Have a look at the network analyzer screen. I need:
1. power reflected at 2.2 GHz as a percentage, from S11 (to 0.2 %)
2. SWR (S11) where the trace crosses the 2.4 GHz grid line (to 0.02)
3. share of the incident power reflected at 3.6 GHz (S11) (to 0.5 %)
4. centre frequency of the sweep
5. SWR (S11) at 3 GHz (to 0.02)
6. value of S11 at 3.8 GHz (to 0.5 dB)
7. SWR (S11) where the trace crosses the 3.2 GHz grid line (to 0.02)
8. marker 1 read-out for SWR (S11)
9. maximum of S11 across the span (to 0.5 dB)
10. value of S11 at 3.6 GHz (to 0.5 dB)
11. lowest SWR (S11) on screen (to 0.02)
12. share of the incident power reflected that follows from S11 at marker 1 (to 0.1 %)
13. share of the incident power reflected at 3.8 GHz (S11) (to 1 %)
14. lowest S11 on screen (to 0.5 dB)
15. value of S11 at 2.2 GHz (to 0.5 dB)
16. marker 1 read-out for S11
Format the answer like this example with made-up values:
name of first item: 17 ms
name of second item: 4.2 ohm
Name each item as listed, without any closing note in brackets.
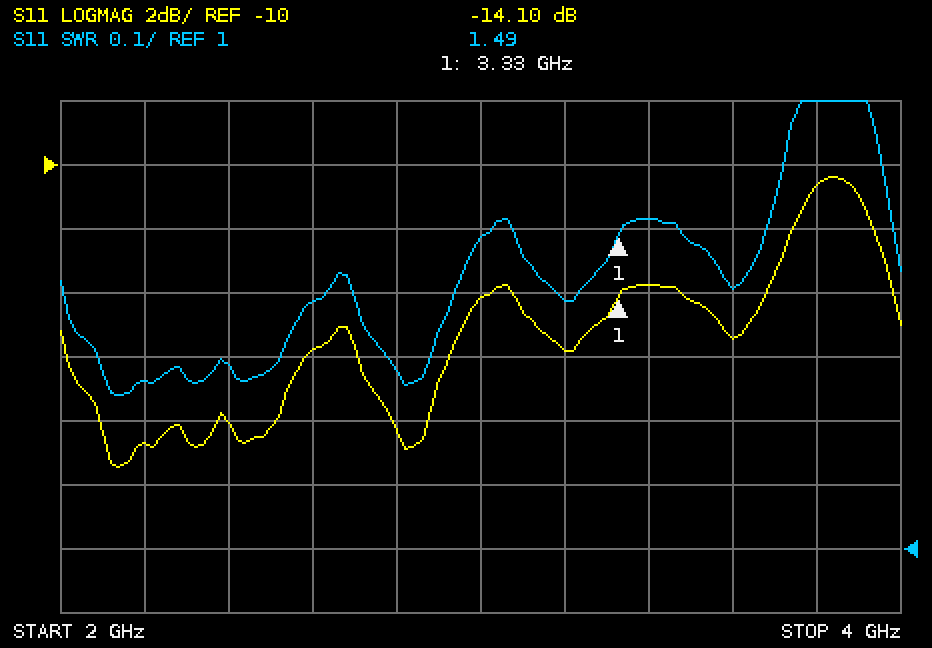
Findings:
power reflected at 2.2 GHz as a percentage, from S11: 1.4 %
SWR (S11) where the trace crosses the 2.4 GHz grid line: 1.28
share of the incident power reflected at 3.6 GHz (S11): 3.0 %
centre frequency of the sweep: 3 GHz
SWR (S11) at 3 GHz: 1.48
value of S11 at 3.8 GHz: -10.5 dB
SWR (S11) where the trace crosses the 3.2 GHz grid line: 1.38
marker 1 read-out for SWR: 1.49
maximum of S11 across the span: -10.5 dB
value of S11 at 3.6 GHz: -15.5 dB
lowest SWR (S11) on screen: 1.24
share of the incident power reflected that follows from S11 at marker 1: 3.9 %
share of the incident power reflected at 3.8 GHz (S11): 9 %
lowest S11 on screen: -19.5 dB
value of S11 at 2.2 GHz: -18.5 dB
marker 1 read-out for S11: -14.10 dB
